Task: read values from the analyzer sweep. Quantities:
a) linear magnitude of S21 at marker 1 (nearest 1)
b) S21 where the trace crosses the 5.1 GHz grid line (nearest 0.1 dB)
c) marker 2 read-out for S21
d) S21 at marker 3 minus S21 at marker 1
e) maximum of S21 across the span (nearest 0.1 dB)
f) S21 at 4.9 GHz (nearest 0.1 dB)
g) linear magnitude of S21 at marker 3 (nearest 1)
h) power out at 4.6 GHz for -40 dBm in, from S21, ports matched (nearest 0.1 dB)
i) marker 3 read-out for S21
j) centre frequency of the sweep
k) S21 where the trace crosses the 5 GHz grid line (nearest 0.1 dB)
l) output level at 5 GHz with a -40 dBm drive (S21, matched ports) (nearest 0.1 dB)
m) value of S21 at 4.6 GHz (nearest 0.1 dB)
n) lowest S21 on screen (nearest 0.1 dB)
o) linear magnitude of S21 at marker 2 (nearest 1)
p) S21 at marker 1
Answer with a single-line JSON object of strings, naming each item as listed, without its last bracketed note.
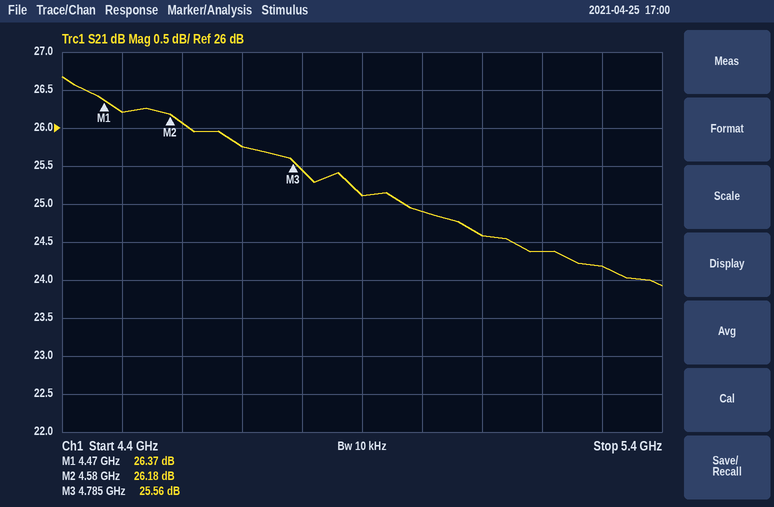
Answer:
{"linear magnitude of S21 at marker 1": "21", "S21 where the trace crosses the 5.1 GHz grid line": "24.6 dB", "marker 2 read-out for S21": "26.18 dB", "S21 at marker 3 minus S21 at marker 1": "-0.81 dB", "maximum of S21 across the span": "26.7 dB", "S21 at 4.9 GHz": "25.1 dB", "linear magnitude of S21 at marker 3": "19", "power out at 4.6 GHz for -40 dBm in, from S21, ports matched": "-13.9 dBm", "marker 3 read-out for S21": "25.56 dB", "centre frequency of the sweep": "4.9 GHz", "S21 where the trace crosses the 5 GHz grid line": "24.9 dB", "output level at 5 GHz with a -40 dBm drive (S21, matched ports)": "-15.1 dBm", "value of S21 at 4.6 GHz": "26.1 dB", "lowest S21 on screen": "23.9 dB", "linear magnitude of S21 at marker 2": "20", "S21 at marker 1": "26.37 dB"}
